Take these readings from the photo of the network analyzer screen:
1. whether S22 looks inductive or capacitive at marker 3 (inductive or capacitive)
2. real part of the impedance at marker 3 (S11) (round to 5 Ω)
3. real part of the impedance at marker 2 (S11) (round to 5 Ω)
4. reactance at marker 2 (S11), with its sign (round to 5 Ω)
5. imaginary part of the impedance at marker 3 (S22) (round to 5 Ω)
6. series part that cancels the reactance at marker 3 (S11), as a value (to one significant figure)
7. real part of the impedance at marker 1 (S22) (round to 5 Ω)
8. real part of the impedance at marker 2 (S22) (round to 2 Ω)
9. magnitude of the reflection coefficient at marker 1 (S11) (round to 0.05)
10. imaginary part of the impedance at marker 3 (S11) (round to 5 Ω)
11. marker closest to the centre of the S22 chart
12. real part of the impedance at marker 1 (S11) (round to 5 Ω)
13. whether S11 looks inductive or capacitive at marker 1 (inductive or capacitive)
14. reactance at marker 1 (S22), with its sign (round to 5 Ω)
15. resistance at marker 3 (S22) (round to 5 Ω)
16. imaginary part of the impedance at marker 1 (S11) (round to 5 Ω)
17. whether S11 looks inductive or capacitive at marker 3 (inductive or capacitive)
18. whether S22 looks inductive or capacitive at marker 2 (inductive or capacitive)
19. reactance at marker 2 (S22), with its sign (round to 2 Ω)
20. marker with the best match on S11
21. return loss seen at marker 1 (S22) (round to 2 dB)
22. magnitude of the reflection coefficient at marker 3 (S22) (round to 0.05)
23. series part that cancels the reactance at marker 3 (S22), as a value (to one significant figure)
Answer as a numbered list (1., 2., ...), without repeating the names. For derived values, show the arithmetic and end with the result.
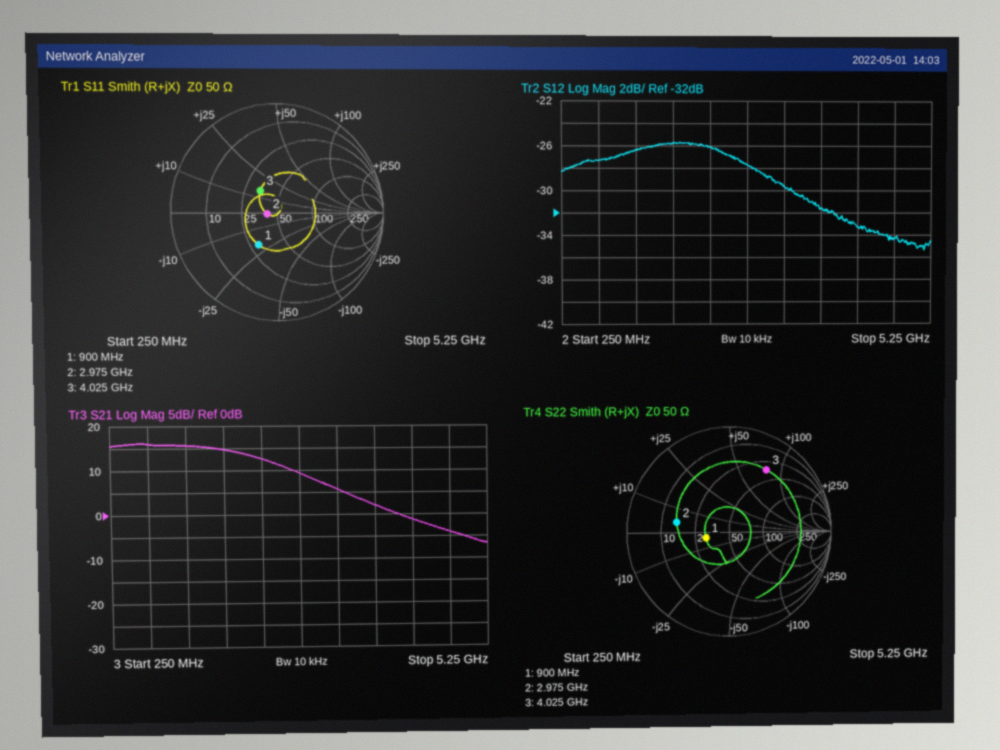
1. inductive
2. 35 Ω
3. 40 Ω
4. 0 Ω
5. +80 Ω
6. C = 1/(2π × 4.025 GHz × 15 Ω) ≈ 3 pF
7. 30 Ω
8. 16 Ω
9. 0.35
10. +15 Ω
11. marker 1
12. 30 Ω
13. capacitive
14. -5 Ω
15. 35 Ω
16. -20 Ω
17. inductive
18. inductive
19. +4 Ω
20. marker 2
21. 12 dB
22. 0.70
23. C = 1/(2π × 4.025 GHz × 80 Ω) ≈ 494 fF, so 500 fF to one significant figure
